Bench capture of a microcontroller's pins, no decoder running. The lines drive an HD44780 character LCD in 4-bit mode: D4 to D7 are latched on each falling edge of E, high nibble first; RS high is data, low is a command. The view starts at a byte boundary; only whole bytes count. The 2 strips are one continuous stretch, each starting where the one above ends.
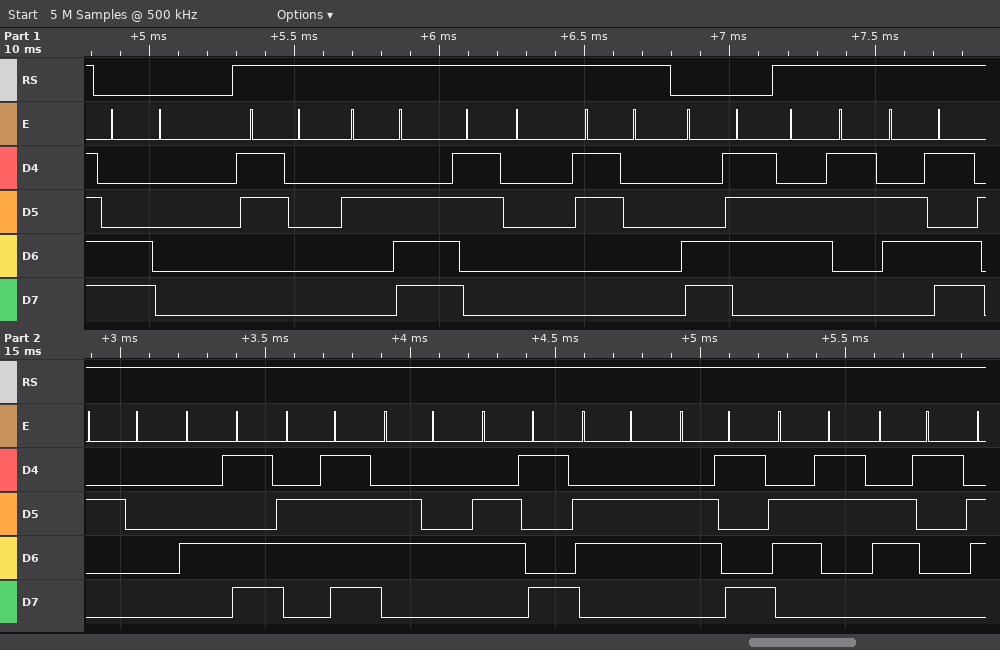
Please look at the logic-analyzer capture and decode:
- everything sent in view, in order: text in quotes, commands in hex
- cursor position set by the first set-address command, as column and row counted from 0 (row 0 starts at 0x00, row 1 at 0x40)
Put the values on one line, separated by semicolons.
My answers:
0xC0 "0.00" 0xC7 "cm Modifica"; column 0, row 1
